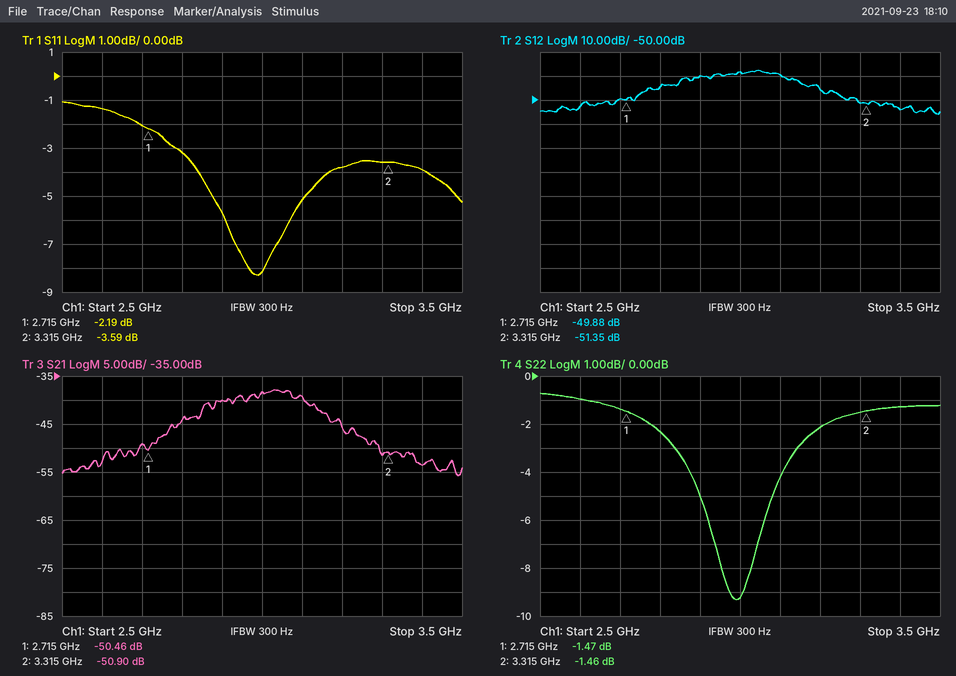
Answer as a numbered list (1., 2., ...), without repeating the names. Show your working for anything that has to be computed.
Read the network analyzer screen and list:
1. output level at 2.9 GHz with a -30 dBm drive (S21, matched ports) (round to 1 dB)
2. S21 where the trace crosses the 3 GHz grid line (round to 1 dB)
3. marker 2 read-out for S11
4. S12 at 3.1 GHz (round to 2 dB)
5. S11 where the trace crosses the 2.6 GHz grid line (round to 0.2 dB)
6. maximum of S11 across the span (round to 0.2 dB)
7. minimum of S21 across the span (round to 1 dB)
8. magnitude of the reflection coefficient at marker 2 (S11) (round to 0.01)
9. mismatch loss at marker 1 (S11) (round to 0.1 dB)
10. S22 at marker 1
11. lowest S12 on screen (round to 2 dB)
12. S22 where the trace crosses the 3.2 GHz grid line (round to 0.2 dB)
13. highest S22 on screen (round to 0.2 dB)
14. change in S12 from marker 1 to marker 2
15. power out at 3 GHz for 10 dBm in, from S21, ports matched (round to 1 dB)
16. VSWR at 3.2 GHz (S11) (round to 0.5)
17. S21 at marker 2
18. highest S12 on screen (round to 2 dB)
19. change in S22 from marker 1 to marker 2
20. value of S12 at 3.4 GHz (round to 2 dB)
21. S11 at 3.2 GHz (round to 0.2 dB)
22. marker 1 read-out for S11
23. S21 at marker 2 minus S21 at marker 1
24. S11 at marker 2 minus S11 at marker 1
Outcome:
1. -30 dBm + (-40 dB) = -70 dBm
2. -38 dB
3. -3.59 dB
4. -40 dB
5. -1.4 dB
6. -1.0 dB
7. -56 dB
8. 10^(-3.59/20) ≈ 0.66
9. −10 log10(1 − 10^(-2.19/10)) ≈ 4.0 dB
10. -1.47 dB
11. -56 dB
12. -2.2 dB
13. -0.8 dB
14. -51.35 − (-49.88) = -1.47 dB
15. 10 dBm + (-38 dB) = -28 dBm
16. |Γ| = 10^(-3.8/20) = 0.6457; VSWR = (1 + 0.6457)/(1 − 0.6457) ≈ 4.64, so 4.5 to the nearest 0.5
17. -50.90 dB
18. -38 dB
19. -1.46 − (-1.47) = 0.01 dB
20. -54 dB
21. -3.8 dB
22. -2.19 dB
23. -50.9 − (-50.46) = -0.44 dB
24. -3.59 − (-2.19) = -1.40 dB
